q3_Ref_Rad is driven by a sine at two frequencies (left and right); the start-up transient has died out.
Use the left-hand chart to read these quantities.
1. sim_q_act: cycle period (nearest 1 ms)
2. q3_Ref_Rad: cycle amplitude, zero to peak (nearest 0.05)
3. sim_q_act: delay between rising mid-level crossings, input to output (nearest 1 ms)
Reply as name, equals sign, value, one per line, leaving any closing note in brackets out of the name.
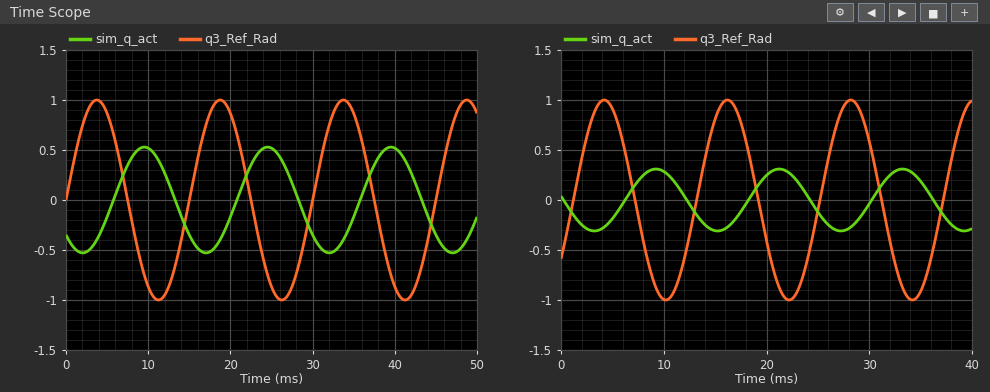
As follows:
sim_q_act: cycle period = 15 ms
q3_Ref_Rad: cycle amplitude, zero to peak = 1.00
sim_q_act: delay between rising mid-level crossings, input to output = 6 ms
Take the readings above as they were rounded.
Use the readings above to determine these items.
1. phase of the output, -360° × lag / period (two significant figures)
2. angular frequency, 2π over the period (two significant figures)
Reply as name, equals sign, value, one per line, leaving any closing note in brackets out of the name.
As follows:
phase of the output, -360° × lag / period = -140°
angular frequency, 2π over the period = 0.42 rad/ms
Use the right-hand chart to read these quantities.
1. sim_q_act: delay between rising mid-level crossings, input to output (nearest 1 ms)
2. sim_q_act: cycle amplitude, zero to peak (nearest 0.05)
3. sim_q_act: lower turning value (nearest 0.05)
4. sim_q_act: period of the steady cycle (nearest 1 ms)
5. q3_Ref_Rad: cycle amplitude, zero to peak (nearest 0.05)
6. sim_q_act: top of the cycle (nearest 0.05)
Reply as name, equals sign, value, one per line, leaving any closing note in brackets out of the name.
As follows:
sim_q_act: delay between rising mid-level crossings, input to output = 5 ms
sim_q_act: cycle amplitude, zero to peak = 0.30
sim_q_act: lower turning value = -0.30
sim_q_act: period of the steady cycle = 12 ms
q3_Ref_Rad: cycle amplitude, zero to peak = 1.00
sim_q_act: top of the cycle = 0.30
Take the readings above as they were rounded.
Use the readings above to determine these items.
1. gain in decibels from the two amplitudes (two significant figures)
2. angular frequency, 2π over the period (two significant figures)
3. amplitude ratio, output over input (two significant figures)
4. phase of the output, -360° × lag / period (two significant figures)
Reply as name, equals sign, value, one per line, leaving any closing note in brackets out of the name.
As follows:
gain in decibels from the two amplitudes = -10 dB
angular frequency, 2π over the period = 0.52 rad/ms
amplitude ratio, output over input = 0.30
phase of the output, -360° × lag / period = -150°
